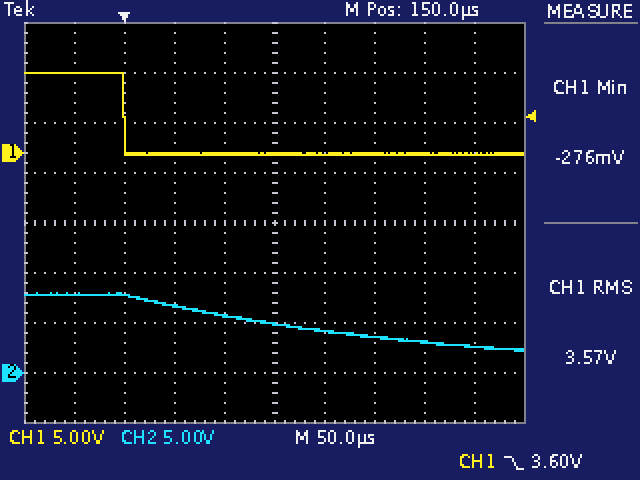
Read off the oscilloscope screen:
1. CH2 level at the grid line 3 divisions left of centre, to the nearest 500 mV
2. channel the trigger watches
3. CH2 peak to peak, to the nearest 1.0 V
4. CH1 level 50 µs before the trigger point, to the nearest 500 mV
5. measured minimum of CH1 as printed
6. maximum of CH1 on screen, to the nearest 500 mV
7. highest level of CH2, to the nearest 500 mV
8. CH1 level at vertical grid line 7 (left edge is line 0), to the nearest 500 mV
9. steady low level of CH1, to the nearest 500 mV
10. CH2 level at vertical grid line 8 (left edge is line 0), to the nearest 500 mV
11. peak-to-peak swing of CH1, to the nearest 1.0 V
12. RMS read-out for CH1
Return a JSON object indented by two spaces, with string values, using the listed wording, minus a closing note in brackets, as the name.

{
  "CH2 level at the grid line 3 divisions left of centre, to the nearest 500 mV": "8.0 V",
  "channel the trigger watches": "CH1",
  "CH2 peak to peak, to the nearest 1.0 V": "6.0 V",
  "CH1 level 50 µs before the trigger point, to the nearest 500 mV": "8.0 V",
  "measured minimum of CH1 as printed": "-276 mV",
  "maximum of CH1 on screen, to the nearest 500 mV": "8.0 V",
  "highest level of CH2, to the nearest 500 mV": "8.0 V",
  "CH1 level at vertical grid line 7 (left edge is line 0), to the nearest 500 mV": "0.0 V",
  "steady low level of CH1, to the nearest 500 mV": "0.0 V",
  "CH2 level at vertical grid line 8 (left edge is line 0), to the nearest 500 mV": "3.0 V",
  "peak-to-peak swing of CH1, to the nearest 1.0 V": "8.0 V",
  "RMS read-out for CH1": "3.57 V"
}
